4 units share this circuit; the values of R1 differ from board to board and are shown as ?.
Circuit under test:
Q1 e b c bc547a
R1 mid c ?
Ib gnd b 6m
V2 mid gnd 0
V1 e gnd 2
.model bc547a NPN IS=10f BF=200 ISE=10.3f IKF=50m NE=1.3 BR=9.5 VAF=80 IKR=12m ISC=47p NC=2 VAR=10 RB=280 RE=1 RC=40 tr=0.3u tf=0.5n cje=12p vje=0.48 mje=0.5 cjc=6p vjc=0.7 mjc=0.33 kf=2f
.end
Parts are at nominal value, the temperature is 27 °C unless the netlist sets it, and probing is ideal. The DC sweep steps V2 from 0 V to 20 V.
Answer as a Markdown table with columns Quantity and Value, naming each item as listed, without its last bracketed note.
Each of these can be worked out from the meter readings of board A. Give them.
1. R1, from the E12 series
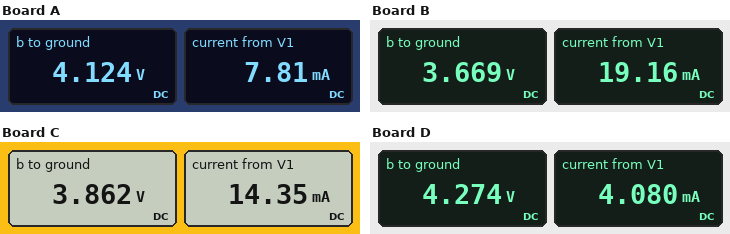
| Quantity | Value |
|---|---|
| R1, from the E12 series | 120 Ω |
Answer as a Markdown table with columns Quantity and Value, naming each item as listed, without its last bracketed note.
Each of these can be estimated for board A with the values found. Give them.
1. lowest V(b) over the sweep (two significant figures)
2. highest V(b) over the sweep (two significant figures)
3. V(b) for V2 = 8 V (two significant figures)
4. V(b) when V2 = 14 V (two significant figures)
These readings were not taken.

| Quantity | Value |
|---|---|
| lowest V(b) over the sweep | 4.1 V |
| highest V(b) over the sweep | 6.3 V |
| V(b) for V2 = 8 V | 5.6 V |
| V(b) when V2 = 14 V | 6.0 V |
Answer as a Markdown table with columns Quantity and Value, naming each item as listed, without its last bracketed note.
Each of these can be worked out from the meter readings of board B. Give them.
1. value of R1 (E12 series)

| Quantity | Value |
|---|---|
| value of R1 | 47 Ω |
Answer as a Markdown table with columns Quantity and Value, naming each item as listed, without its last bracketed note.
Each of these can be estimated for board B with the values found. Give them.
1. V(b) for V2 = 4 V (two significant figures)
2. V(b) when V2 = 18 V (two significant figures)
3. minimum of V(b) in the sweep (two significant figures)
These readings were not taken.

| Quantity | Value |
|---|---|
| V(b) for V2 = 4 V | 5.4 V |
| V(b) when V2 = 18 V | 6.4 V |
| minimum of V(b) in the sweep | 3.7 V |
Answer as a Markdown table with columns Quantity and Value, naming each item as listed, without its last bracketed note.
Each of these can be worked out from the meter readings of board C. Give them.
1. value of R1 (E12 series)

| Quantity | Value |
|---|---|
| value of R1 | 68 Ω |
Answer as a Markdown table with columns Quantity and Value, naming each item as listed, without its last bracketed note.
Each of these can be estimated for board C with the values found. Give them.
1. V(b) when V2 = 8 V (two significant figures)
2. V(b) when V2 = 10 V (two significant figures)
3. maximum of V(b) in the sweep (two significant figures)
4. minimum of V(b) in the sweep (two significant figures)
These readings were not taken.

| Quantity | Value |
|---|---|
| V(b) when V2 = 8 V | 5.7 V |
| V(b) when V2 = 10 V | 5.8 V |
| maximum of V(b) in the sweep | 6.5 V |
| minimum of V(b) in the sweep | 3.9 V |
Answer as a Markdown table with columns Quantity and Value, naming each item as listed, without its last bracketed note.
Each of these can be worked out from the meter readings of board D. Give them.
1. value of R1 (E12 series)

| Quantity | Value |
|---|---|
| value of R1 | 180 Ω |
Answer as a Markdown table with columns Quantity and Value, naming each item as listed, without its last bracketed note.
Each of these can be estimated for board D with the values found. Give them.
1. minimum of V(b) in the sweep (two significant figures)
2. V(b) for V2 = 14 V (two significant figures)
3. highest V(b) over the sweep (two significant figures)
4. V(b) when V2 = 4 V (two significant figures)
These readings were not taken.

| Quantity | Value |
|---|---|
| minimum of V(b) in the sweep | 4.3 V |
| V(b) for V2 = 14 V | 5.9 V |
| highest V(b) over the sweep | 6.2 V |
| V(b) when V2 = 4 V | 5.0 V |
